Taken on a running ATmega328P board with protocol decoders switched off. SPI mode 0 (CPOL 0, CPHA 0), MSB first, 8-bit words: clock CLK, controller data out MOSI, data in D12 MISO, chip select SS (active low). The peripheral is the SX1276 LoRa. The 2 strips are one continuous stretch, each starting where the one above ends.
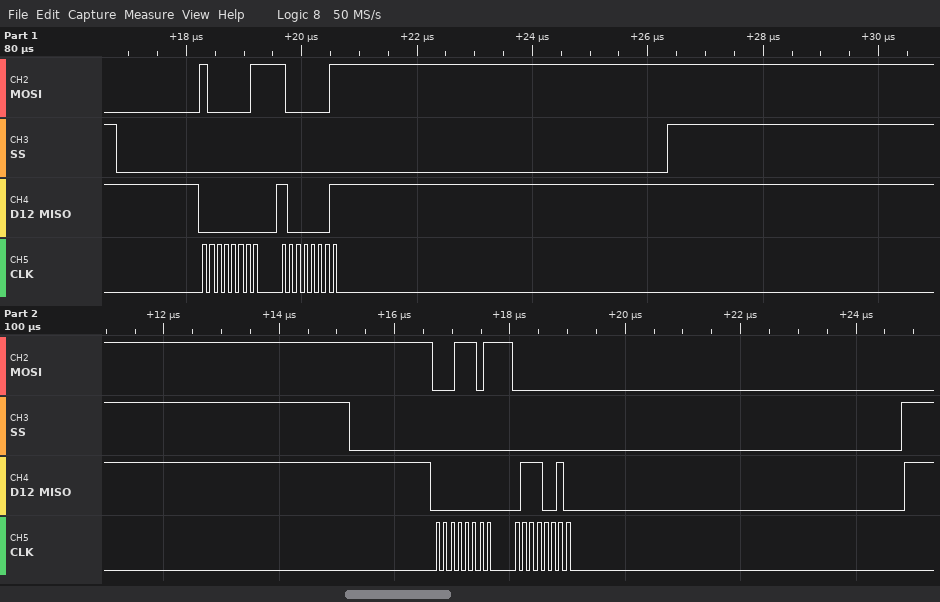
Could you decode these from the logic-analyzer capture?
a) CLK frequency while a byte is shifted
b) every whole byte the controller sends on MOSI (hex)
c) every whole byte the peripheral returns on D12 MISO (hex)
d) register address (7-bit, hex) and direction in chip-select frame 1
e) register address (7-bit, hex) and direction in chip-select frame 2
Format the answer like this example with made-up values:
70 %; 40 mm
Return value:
8 MHz; 0x81 0x81 0x1D 0x00; 0x00 0x81 0x00 0x72; 0x01 write; 0x1D read
